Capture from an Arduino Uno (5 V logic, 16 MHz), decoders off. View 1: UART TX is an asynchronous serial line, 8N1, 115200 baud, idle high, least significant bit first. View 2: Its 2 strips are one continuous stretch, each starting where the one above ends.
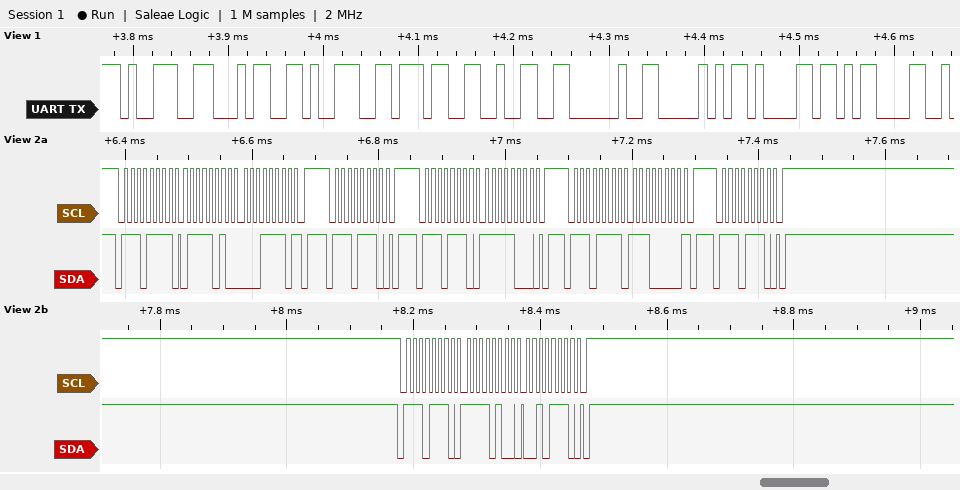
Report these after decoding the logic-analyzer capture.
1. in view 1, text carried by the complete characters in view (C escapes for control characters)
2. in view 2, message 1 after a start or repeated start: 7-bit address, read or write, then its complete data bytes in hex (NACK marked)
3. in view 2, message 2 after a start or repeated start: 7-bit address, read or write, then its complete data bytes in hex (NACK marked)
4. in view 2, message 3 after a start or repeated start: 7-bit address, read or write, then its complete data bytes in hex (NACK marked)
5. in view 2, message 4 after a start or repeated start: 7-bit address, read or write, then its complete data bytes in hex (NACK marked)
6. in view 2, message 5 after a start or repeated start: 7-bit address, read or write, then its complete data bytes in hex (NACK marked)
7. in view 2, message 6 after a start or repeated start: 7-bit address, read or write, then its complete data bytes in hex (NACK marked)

"94972 Pa\r"
0x77 read: 7A 1E NACK
0x77 write
0x77 write: F8
0x77 read: E0 NACK
0x77 write
0x77 write: F4 2E
